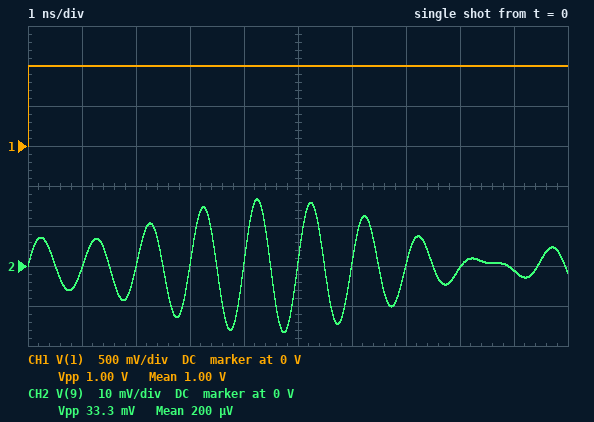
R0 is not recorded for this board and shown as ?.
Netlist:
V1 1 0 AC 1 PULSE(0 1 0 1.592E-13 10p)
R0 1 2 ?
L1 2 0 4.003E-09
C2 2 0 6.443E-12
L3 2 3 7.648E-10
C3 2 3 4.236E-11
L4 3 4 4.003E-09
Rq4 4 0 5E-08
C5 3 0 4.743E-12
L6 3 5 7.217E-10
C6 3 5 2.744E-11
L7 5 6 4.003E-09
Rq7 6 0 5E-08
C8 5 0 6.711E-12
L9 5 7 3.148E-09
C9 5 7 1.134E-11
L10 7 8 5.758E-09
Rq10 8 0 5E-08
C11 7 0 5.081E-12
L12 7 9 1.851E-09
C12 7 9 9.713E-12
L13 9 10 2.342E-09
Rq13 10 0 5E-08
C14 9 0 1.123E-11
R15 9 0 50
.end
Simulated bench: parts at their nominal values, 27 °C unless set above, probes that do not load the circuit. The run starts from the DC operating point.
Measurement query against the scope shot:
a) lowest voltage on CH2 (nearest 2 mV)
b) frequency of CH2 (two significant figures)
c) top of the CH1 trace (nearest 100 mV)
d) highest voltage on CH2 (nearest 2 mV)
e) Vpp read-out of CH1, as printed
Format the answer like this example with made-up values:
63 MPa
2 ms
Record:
-16 mV
1.0 GHz
1.0 V
16 mV
1.00 V
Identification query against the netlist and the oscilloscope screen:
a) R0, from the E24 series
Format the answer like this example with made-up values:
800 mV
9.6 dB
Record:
150 Ω
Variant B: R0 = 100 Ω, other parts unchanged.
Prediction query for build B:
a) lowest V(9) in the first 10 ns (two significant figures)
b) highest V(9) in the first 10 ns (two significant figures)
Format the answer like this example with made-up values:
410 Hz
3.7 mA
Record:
-22 mV
22 mV
